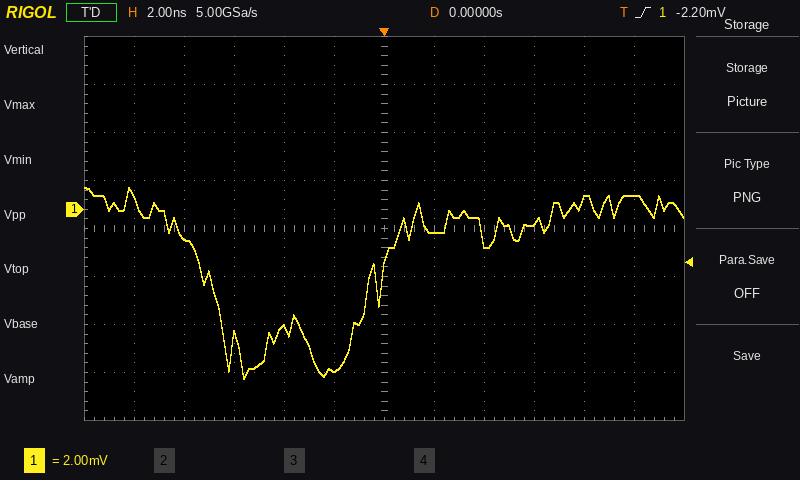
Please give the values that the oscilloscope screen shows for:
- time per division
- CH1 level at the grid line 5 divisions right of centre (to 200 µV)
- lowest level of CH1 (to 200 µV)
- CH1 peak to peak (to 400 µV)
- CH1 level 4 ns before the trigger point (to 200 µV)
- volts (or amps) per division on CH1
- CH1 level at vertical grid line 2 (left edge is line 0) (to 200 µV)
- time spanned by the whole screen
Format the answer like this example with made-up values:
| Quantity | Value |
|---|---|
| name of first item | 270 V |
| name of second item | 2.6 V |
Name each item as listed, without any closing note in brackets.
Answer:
| Quantity | Value |
|---|---|
| time per division | 2 ns |
| CH1 level at the grid line 5 divisions right of centre | 600 µV |
| lowest level of CH1 | -7.0 mV |
| CH1 peak to peak | 8.0 mV |
| CH1 level 4 ns before the trigger point | -5.0 mV |
| volts (or amps) per division on CH1 | 2 mV |
| CH1 level at vertical grid line 2 (left edge is line 0) | -1.2 mV |
| time spanned by the whole screen | 24 ns |
